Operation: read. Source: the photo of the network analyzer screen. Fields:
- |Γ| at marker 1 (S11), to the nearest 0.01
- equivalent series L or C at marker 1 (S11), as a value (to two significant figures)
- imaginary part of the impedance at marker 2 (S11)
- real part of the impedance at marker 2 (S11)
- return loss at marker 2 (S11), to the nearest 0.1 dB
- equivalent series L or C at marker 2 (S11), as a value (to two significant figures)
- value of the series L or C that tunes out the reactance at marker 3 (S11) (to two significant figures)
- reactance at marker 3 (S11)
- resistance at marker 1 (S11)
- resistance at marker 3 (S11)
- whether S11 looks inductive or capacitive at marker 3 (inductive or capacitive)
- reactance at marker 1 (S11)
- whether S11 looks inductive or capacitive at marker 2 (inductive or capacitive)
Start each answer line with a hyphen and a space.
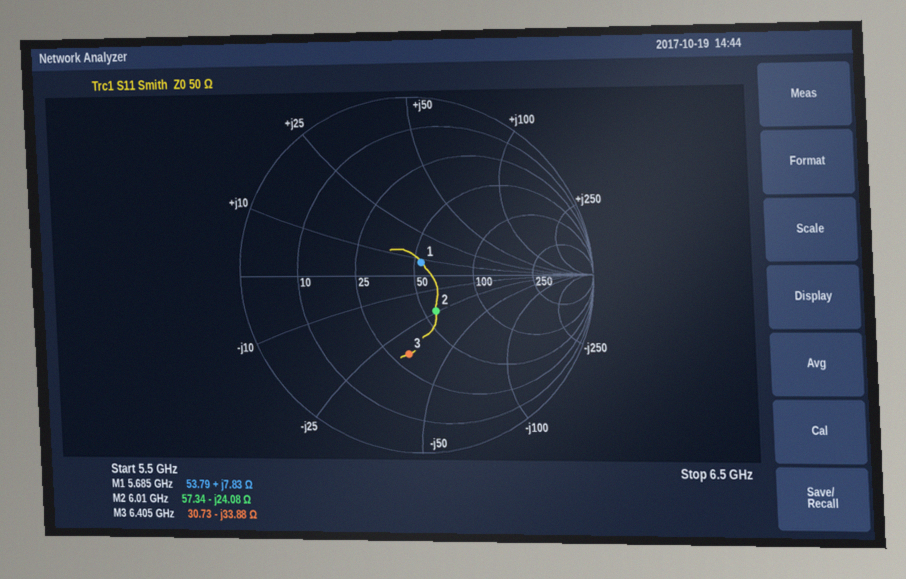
- 0.08
- 220 pH
- -24.08 Ω
- 57.34 Ω
- 12.8 dB
- 1.1 pF
- 840 pH
- -33.88 Ω
- 53.79 Ω
- 30.73 Ω
- capacitive
- +7.83 Ω
- capacitive
